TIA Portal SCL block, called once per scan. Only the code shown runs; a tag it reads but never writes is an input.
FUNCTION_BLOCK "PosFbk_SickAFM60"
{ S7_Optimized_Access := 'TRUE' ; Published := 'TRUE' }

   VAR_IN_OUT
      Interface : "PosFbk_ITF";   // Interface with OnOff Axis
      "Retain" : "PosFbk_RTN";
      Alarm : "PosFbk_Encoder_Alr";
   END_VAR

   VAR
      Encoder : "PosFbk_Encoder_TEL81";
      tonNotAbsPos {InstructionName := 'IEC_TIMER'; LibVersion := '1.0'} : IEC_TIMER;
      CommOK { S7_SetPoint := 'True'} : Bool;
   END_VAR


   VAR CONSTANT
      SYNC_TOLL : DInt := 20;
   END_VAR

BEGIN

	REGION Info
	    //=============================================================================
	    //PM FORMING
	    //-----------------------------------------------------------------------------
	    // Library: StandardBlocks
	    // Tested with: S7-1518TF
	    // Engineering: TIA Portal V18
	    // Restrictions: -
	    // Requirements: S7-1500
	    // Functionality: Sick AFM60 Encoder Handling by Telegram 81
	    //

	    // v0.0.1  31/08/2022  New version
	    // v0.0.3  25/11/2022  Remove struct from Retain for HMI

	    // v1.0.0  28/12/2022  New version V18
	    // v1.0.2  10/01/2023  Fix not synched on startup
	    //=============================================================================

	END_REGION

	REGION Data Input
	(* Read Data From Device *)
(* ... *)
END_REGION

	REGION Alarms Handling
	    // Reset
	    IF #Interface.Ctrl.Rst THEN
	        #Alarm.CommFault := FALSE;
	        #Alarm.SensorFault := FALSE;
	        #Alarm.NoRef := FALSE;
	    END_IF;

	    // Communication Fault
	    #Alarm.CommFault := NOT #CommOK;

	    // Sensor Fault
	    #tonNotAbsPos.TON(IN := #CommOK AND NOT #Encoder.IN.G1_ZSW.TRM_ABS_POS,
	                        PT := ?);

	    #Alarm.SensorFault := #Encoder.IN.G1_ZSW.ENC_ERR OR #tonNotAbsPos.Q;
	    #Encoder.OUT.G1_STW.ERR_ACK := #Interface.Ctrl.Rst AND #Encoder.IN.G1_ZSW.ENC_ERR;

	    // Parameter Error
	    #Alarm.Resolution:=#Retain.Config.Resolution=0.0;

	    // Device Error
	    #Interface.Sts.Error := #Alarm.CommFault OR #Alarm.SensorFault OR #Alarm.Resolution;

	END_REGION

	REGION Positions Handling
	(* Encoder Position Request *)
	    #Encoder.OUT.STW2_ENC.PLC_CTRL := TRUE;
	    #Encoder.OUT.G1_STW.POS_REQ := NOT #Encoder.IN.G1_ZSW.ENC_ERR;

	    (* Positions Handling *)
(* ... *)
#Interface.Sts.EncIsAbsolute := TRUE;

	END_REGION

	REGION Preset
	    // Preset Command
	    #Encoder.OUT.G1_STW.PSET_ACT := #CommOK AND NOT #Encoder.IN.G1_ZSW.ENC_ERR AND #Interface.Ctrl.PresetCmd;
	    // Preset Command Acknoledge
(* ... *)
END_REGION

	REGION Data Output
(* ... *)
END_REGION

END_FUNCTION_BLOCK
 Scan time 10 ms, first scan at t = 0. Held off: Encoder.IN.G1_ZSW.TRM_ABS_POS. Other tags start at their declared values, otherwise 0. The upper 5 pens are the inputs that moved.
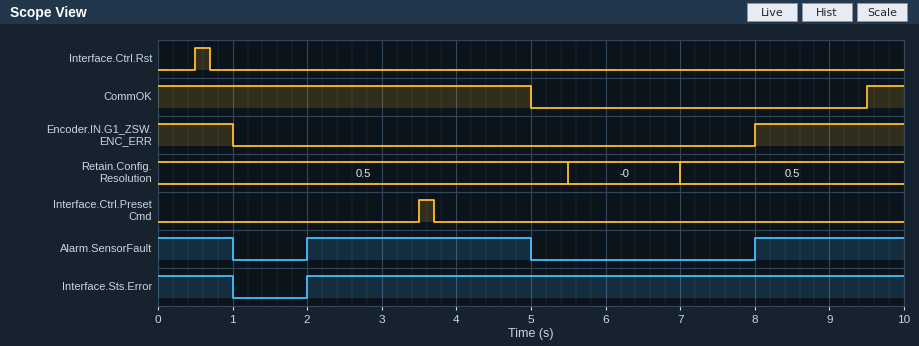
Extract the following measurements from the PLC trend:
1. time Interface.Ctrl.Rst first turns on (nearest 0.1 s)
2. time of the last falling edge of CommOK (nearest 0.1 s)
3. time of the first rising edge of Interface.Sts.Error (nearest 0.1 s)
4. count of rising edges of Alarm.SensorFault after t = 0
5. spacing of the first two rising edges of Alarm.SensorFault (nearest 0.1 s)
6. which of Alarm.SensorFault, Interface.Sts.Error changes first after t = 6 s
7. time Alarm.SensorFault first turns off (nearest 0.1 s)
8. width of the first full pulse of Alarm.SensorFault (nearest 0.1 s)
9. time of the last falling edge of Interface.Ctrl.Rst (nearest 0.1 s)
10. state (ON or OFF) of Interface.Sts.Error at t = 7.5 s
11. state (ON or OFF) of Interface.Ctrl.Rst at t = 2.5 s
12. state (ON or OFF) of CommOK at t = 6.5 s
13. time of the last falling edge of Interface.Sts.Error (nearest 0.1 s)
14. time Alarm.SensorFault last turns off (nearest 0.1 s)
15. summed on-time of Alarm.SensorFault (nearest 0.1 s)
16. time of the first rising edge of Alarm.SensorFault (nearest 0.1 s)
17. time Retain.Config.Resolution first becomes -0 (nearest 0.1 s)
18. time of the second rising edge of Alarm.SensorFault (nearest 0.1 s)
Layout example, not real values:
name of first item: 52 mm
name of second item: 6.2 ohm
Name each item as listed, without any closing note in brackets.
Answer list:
time Interface.Ctrl.Rst first turns on: 0.5 s
time of the last falling edge of CommOK: 5.0 s
time of the first rising edge of Interface.Sts.Error: 2.0 s
count of rising edges of Alarm.SensorFault after t = 0: 2
spacing of the first two rising edges of Alarm.SensorFault: 6.0 s
which of Alarm.SensorFault, Interface.Sts.Error changes first after t = 6 s: Alarm.SensorFault
time Alarm.SensorFault first turns off: 1.0 s
width of the first full pulse of Alarm.SensorFault: 3.0 s
time of the last falling edge of Interface.Ctrl.Rst: 0.7 s
state (ON or OFF) of Interface.Sts.Error at t = 7.5 s: ON
state (ON or OFF) of Interface.Ctrl.Rst at t = 2.5 s: OFF
state (ON or OFF) of CommOK at t = 6.5 s: OFF
time of the last falling edge of Interface.Sts.Error: 1.0 s
time Alarm.SensorFault last turns off: 5.0 s
summed on-time of Alarm.SensorFault: 6.0 s
time of the first rising edge of Alarm.SensorFault: 2.0 s
time Retain.Config.Resolution first becomes -0: 5.5 s
time of the second rising edge of Alarm.SensorFault: 8.0 s
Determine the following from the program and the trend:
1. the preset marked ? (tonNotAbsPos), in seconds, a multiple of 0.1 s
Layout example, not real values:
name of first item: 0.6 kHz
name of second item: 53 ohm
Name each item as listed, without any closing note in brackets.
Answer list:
the preset marked ? (tonNotAbsPos), in seconds, a multiple of 0.1 s: 2.0 s
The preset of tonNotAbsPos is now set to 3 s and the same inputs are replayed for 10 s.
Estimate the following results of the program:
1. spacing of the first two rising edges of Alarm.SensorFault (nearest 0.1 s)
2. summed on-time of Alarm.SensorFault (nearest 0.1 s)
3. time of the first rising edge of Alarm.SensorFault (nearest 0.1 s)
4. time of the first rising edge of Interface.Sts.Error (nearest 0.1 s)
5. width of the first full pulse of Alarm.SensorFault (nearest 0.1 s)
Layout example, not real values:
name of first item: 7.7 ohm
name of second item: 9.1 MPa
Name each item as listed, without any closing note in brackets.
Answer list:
spacing of the first two rising edges of Alarm.SensorFault: 5.0 s
summed on-time of Alarm.SensorFault: 5.0 s
time of the first rising edge of Alarm.SensorFault: 3.0 s
time of the first rising edge of Interface.Sts.Error: 3.0 s
width of the first full pulse of Alarm.SensorFault: 2.0 s
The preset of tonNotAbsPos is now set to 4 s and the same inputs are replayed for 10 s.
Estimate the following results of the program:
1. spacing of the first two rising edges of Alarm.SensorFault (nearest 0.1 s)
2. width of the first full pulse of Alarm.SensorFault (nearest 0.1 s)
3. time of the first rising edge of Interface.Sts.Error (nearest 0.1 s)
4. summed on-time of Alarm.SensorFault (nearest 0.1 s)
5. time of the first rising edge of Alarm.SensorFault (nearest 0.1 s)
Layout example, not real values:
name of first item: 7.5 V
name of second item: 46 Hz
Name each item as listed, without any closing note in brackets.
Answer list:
spacing of the first two rising edges of Alarm.SensorFault: 4.0 s
width of the first full pulse of Alarm.SensorFault: 1.0 s
time of the first rising edge of Interface.Sts.Error: 4.0 s
summed on-time of Alarm.SensorFault: 4.0 s
time of the first rising edge of Alarm.SensorFault: 4.0 s
